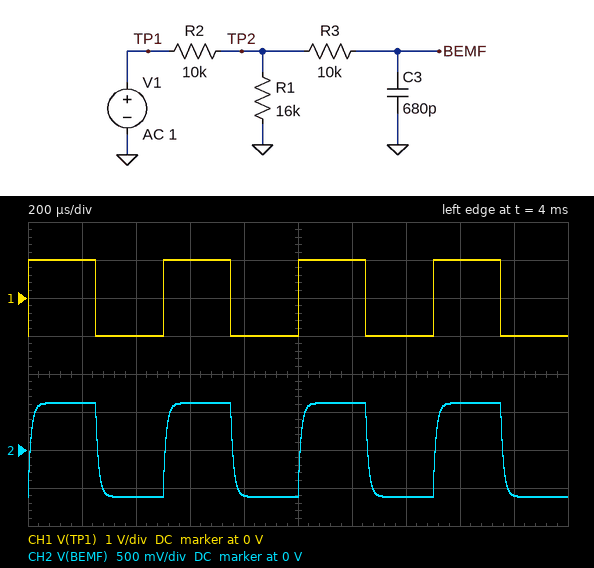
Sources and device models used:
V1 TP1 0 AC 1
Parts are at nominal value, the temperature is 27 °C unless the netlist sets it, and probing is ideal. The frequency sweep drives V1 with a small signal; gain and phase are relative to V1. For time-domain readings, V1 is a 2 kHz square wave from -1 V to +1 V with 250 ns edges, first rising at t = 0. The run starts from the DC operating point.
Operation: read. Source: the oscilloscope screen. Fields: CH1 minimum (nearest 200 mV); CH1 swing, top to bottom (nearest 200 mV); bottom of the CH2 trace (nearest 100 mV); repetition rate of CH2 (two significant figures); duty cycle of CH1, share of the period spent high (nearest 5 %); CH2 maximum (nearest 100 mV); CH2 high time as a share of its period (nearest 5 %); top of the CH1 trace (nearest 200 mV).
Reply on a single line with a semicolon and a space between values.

-1.0 V; 2.0 V; -600 mV; 2.0 kHz; 50 %; 600 mV; 50 %; 1.0 V
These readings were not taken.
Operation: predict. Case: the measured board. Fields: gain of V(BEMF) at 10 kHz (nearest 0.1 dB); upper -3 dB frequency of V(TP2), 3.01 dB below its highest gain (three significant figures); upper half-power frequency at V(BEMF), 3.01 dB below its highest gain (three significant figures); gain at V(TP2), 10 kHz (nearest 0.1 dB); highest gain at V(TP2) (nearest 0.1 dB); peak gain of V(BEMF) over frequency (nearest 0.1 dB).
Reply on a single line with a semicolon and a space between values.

-5.9 dB; 30.0 kHz; 14.5 kHz; -5.2 dB; -4.2 dB; -4.2 dB
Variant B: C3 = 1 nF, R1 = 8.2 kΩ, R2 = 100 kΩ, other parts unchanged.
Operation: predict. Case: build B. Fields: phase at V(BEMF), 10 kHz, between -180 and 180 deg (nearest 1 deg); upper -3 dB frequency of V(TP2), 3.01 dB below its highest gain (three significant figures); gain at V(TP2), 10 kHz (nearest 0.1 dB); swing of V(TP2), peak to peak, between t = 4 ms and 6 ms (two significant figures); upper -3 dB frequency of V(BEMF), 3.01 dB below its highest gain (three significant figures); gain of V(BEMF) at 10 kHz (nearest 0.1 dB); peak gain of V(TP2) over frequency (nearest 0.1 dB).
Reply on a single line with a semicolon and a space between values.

-48 deg; 15.2 kHz; -24.4 dB; 150 mV; 9.05 kHz; -25.9 dB; -22.4 dB
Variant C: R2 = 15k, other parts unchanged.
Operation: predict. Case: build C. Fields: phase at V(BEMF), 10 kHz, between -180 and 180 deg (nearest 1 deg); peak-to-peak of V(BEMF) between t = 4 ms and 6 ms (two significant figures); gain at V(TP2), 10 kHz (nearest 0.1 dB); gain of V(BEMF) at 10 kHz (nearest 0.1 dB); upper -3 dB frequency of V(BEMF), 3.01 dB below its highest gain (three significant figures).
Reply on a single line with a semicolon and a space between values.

-37 deg; 1.0 V; -7.0 dB; -7.7 dB; 13.2 kHz
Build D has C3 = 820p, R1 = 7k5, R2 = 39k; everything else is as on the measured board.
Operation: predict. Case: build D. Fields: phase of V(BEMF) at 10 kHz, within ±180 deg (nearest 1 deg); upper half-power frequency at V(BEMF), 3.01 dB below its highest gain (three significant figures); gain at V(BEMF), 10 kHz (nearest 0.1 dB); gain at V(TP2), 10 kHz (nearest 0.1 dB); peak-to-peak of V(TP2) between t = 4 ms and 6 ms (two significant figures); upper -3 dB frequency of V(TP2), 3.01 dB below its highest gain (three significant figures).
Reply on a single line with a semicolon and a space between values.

-40 deg; 11.9 kHz; -18.2 dB; -17.1 dB; 320 mV; 24.0 kHz
